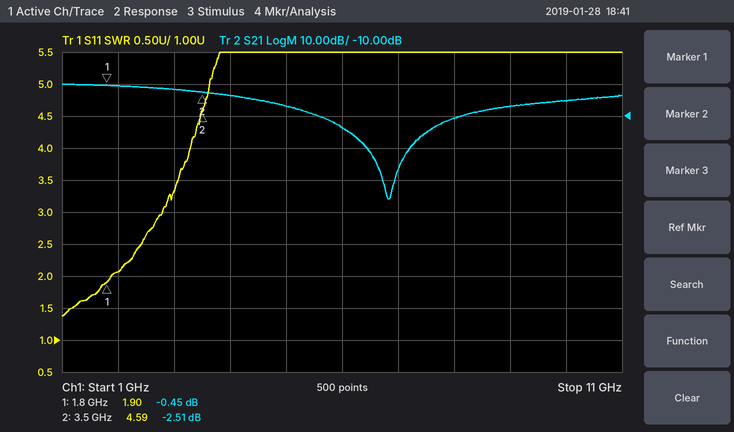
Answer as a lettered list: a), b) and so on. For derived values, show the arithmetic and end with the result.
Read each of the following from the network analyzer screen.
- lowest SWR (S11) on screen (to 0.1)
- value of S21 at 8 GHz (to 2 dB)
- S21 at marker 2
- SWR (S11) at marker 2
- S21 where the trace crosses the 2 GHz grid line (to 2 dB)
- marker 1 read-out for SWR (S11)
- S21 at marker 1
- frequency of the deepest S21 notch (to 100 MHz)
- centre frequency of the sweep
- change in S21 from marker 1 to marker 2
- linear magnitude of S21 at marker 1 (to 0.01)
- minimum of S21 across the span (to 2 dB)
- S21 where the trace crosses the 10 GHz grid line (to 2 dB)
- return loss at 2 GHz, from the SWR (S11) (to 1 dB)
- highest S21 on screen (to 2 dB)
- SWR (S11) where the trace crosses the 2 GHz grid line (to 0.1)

a) 1.4
b) -10 dB
c) -2.51 dB
d) 4.59
e) 0 dB
f) 1.90
g) -0.45 dB
h) 6.8 GHz
i) 6 GHz
j) -2.51 − (-0.45) = -2.06 dB
k) 10^(-0.45/20) ≈ 0.95
l) -36 dB
m) -6 dB
n) −20 log10((2.1 − 1)/(2.1 + 1)) ≈ 9 dB
o) 0 dB
p) 2.1
